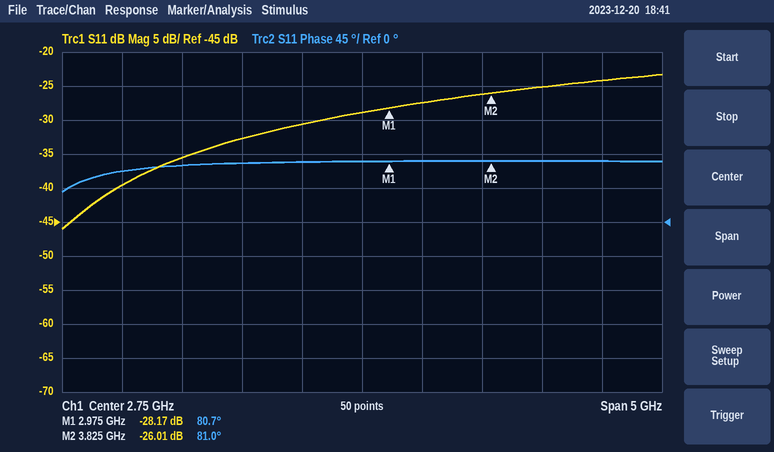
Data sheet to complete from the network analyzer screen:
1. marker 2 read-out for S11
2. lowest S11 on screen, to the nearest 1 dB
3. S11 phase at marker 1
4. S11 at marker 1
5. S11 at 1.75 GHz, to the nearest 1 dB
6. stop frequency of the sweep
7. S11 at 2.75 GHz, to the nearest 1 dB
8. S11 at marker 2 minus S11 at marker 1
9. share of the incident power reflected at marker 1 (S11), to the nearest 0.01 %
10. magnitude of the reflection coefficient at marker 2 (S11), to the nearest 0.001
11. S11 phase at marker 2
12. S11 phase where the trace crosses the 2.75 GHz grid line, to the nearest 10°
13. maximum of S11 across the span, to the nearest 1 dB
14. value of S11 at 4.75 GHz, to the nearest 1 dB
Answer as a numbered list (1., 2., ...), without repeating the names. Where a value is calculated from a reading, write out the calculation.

1. -26.01 dB
2. -46 dB
3. 80.7°
4. -28.17 dB
5. -33 dB
6. 5.25 GHz
7. -29 dB
8. -26.01 − (-28.17) = 2.16 dB
9. 10^(-28.17/10) ≈ 0.15 %
10. 10^(-26.01/20) ≈ 0.050
11. 81.0°
12. 80°
13. -23 dB
14. -24 dB
